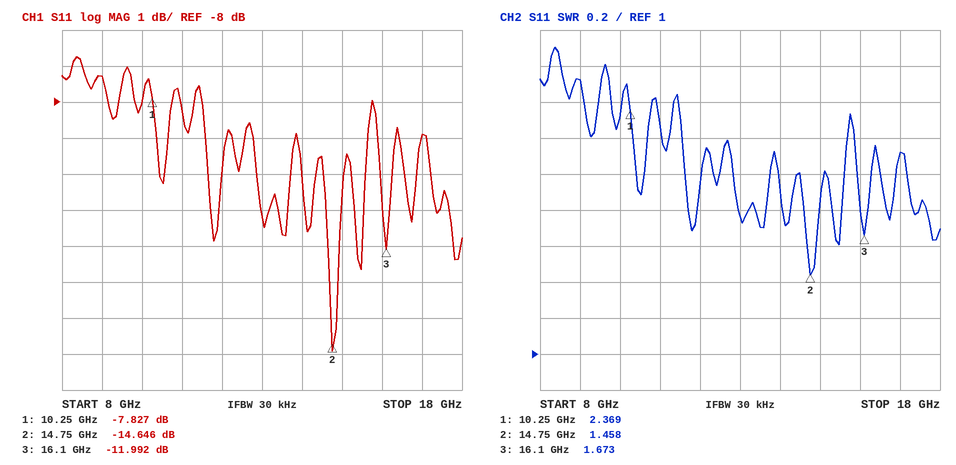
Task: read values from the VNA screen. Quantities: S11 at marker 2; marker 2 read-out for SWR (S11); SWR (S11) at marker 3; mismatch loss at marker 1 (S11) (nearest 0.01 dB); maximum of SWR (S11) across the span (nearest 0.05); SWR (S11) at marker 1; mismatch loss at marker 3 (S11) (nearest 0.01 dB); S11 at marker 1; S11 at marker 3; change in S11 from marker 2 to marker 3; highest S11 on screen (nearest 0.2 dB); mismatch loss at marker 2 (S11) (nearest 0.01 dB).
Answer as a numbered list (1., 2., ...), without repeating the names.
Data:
1. -14.646 dB
2. 1.458
3. 1.673
4. 0.78 dB
5. 2.70
6. 2.369
7. 0.28 dB
8. -7.827 dB
9. -11.992 dB
10. 2.654 dB
11. -6.8 dB
12. 0.15 dB
